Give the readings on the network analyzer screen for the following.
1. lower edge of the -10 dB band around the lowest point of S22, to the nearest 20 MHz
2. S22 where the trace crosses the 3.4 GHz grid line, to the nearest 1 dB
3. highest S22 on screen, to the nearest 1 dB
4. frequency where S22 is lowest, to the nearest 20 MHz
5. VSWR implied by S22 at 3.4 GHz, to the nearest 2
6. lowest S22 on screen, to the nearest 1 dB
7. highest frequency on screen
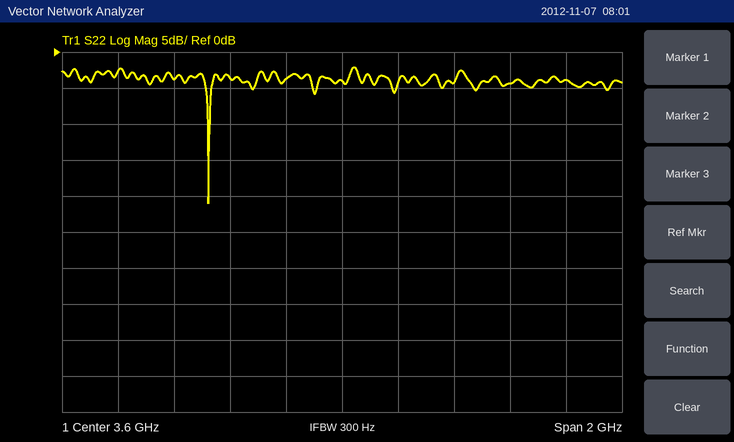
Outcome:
3.12 GHz
-4 dB
-2 dB
3.12 GHz
4
-21 dB
4.6 GHz
